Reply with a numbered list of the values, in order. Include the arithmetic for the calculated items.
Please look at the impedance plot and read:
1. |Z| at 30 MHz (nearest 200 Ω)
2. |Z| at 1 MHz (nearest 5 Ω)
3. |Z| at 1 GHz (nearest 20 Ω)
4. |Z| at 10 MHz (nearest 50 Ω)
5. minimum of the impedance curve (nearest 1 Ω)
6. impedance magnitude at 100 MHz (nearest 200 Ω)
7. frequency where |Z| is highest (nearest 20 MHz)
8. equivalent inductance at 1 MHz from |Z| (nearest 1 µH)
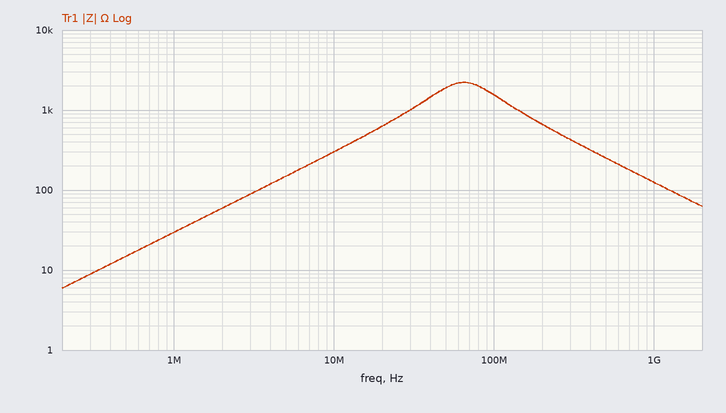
1. 1.0 kΩ
2. 30 Ω
3. 120 Ω
4. 300 Ω
5. 6 Ω
6. 1.6 kΩ
7. 60 MHz
8. L = 30 Ω/(2π × 1 MHz) ≈ 5 µH
